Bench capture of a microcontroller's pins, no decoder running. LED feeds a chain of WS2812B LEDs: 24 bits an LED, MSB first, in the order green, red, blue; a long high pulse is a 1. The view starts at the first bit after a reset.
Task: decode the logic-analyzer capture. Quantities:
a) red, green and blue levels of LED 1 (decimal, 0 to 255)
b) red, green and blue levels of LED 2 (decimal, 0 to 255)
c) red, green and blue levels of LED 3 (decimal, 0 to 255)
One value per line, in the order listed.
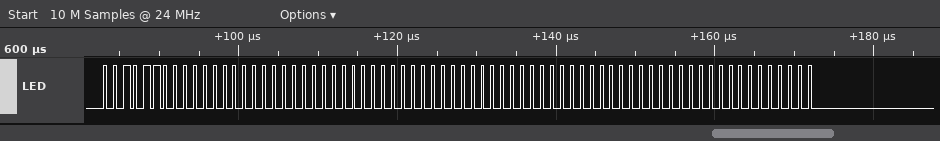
0, 44, 0
0, 0, 0
0, 0, 0
